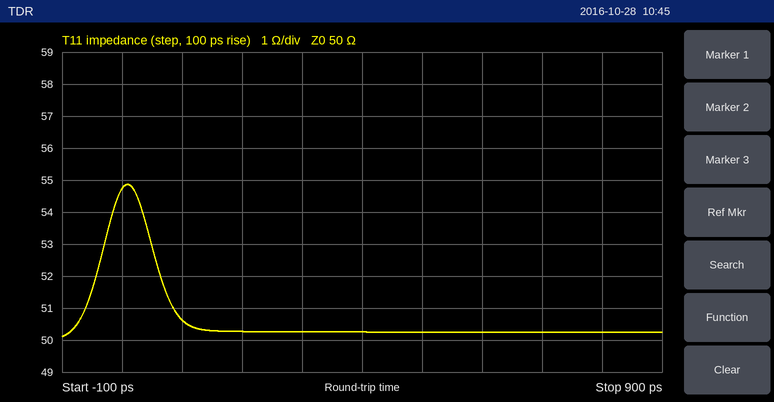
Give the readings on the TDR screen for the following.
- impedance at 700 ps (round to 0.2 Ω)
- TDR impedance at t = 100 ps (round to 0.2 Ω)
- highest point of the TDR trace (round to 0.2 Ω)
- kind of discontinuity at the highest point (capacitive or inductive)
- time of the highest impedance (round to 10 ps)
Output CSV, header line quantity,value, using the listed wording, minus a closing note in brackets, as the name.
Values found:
quantity,value
impedance at 700 ps,50.2 Ω
TDR impedance at t = 100 ps,50.6 Ω
highest point of the TDR trace,54.8 Ω
kind of discontinuity at the highest point,inductive
time of the highest impedance,10 ps
